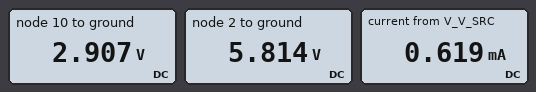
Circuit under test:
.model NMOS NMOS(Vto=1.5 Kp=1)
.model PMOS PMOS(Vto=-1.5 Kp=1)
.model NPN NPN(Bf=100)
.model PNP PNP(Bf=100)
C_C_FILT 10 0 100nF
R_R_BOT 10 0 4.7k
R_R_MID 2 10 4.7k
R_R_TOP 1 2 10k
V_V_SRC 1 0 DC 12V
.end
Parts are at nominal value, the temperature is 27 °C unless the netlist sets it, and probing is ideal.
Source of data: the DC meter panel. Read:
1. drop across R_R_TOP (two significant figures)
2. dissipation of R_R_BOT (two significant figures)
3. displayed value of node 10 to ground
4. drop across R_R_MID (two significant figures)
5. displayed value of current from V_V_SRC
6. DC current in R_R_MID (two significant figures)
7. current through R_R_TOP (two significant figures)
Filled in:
6.2 V
1.8 mW
2.907 V
2.9 V
0.619 mA
620 µA
620 µA
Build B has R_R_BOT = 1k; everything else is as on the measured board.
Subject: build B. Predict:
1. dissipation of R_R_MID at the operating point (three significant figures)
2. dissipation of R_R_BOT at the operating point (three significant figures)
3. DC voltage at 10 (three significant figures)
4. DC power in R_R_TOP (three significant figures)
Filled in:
2.75 mW
584 µW
764 mV
5.84 mW
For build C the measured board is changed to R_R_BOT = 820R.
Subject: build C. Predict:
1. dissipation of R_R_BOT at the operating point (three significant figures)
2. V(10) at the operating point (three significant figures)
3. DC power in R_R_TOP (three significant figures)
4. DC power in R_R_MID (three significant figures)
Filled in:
490 µW
634 mV
5.98 mW
2.81 mW
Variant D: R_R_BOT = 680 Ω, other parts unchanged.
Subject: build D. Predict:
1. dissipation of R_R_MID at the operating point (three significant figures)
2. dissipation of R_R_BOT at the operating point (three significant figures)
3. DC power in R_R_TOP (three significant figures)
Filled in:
2.86 mW
414 µW
6.09 mW
